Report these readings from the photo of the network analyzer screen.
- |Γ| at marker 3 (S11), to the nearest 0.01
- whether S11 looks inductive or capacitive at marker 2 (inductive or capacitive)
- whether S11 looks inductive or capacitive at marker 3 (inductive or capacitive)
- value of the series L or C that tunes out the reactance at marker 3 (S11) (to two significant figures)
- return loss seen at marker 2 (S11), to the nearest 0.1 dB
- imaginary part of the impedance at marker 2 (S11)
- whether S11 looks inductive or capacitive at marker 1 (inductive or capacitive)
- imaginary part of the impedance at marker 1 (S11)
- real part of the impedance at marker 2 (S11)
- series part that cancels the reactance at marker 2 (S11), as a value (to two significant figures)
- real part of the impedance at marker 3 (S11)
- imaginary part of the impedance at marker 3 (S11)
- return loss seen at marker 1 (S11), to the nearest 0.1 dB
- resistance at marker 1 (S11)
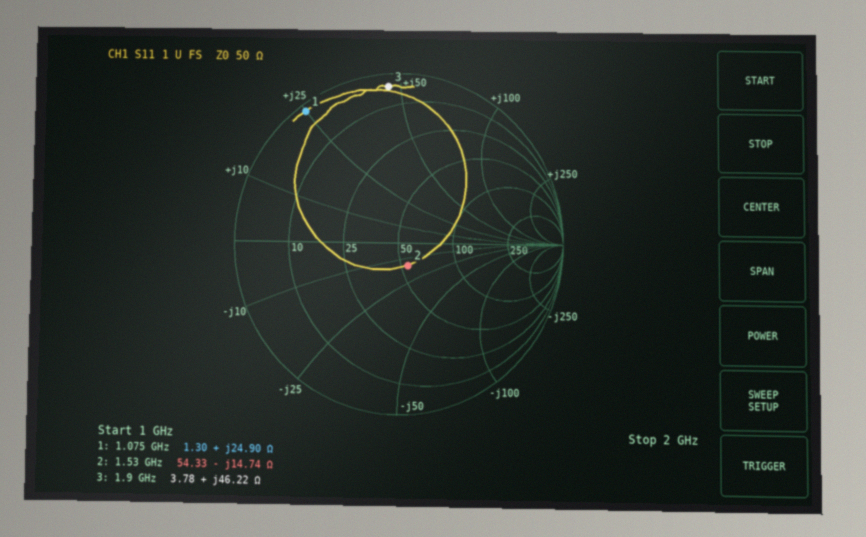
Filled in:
0.92
capacitive
inductive
1.8 pF
16.7 dB
-14.74 Ω
inductive
+24.90 Ω
54.33 Ω
1.5 nH
3.78 Ω
+46.22 Ω
0.4 dB
1.30 Ω
